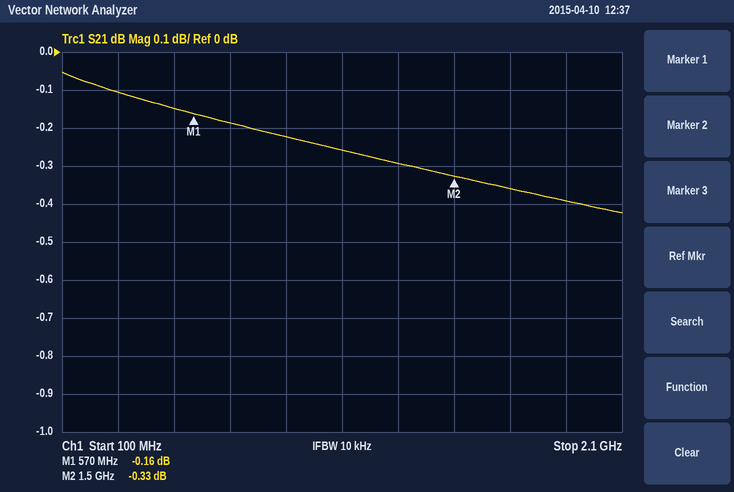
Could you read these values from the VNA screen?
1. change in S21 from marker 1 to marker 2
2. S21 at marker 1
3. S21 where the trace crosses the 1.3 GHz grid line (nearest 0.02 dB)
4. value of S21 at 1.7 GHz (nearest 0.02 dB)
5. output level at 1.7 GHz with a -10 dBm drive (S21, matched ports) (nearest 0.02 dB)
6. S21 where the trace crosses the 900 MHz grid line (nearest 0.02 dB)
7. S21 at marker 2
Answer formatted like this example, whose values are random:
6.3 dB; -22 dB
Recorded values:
-0.17 dB; -0.16 dB; -0.30 dB; -0.36 dB; -10.36 dBm; -0.22 dB; -0.33 dB
